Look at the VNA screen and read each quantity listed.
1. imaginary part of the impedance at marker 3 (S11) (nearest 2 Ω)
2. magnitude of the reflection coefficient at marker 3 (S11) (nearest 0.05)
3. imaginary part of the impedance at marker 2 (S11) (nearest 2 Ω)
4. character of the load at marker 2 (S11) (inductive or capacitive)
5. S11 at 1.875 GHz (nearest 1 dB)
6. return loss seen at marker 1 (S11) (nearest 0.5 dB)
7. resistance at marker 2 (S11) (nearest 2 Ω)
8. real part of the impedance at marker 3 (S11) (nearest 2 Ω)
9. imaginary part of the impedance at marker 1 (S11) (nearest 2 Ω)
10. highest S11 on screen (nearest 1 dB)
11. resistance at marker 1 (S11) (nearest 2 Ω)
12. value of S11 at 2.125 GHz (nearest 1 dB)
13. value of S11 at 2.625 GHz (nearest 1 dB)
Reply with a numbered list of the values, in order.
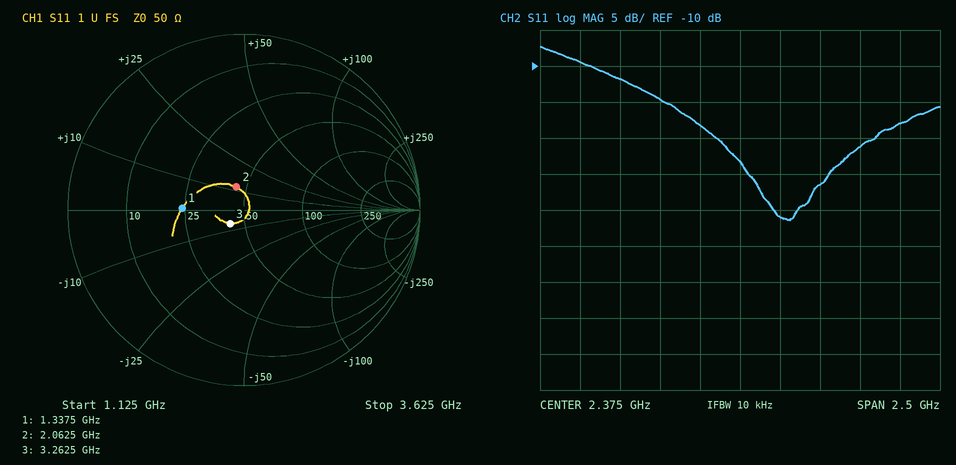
1. -6 Ω
2. 0.10
3. +12 Ω
4. inductive
5. -15 dB
6. 9.0 dB
7. 44 Ω
8. 42 Ω
9. 0 Ω
10. -7 dB
11. 24 Ω
12. -18 dB
13. -31 dB
